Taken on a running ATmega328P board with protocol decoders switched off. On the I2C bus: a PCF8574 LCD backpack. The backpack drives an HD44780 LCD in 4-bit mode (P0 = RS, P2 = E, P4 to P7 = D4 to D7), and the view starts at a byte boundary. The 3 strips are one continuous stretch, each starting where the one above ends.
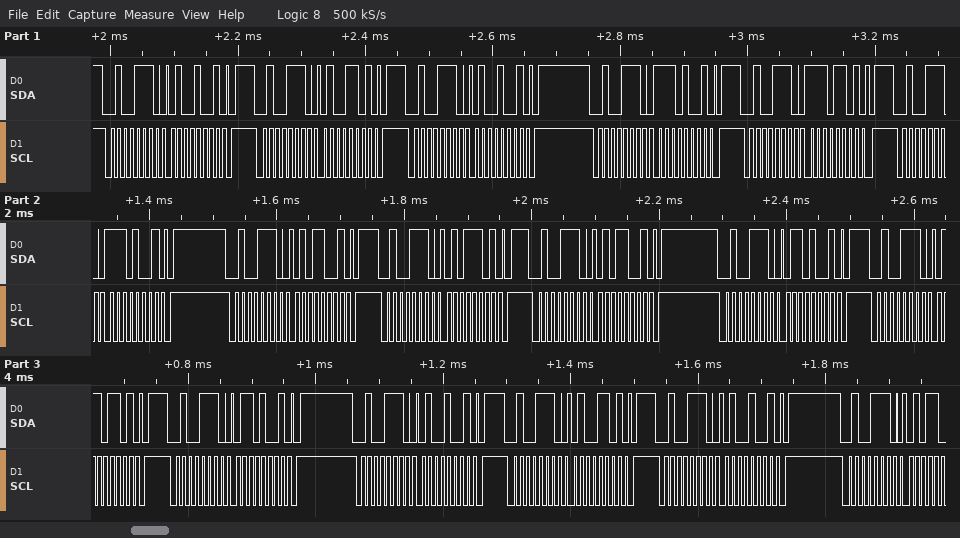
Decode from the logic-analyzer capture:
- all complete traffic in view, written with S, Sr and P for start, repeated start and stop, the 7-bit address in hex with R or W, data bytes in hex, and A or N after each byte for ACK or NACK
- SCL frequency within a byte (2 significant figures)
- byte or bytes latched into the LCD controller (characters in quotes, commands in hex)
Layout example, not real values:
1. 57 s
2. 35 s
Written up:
1. S 27W A 49 A P S 27W A 4D A P S 27W A 49 A P S 27W A E9 A P S 27W A ED A P S 27W A E9 A P S 27W A 59 A P S 27W A 5D A P S 27W A 59 A P S 27W A 69 A P S 27W A 6D A P S 27W A 69 A P S 27W A 49 A P S 27W A 4D A P S 27W A 49 A P S 27W A
2. 100 kHz
3. 'N' 'V'
